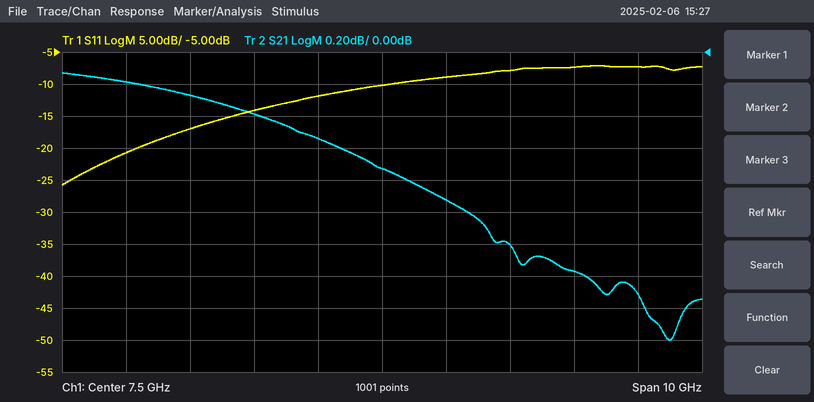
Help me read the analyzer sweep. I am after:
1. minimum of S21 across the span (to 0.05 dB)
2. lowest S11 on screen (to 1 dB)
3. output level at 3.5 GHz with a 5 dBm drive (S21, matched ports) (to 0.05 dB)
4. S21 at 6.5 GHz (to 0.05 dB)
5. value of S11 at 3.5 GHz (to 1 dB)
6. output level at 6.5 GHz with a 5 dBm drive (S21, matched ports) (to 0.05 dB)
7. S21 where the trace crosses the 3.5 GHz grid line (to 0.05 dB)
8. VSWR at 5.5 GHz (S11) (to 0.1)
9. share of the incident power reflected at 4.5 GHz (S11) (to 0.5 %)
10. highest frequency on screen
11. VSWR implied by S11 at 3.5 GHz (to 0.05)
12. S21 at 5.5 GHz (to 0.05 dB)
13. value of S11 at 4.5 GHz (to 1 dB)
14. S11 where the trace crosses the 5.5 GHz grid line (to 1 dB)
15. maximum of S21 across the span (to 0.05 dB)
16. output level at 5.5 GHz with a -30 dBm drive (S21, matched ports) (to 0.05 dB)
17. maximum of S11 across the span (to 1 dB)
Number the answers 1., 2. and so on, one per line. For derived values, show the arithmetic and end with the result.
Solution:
1. -1.80 dB
2. -26 dB
3. 5 dBm + (-0.20 dB) = 4.80 dBm
4. -0.55 dB
5. -21 dB
6. 5 dBm + (-0.55 dB) = 4.45 dBm
7. -0.20 dB
8. |Γ| = 10^(-14/20) = 0.1995; VSWR = (1 + 0.1995)/(1 − 0.1995) ≈ 1.5
9. 10^(-17/10) ≈ 2.0 %
10. 12.5 GHz
11. |Γ| = 10^(-21/20) = 0.0891; VSWR = (1 + 0.0891)/(1 − 0.0891) ≈ 1.20
12. -0.40 dB
13. -17 dB
14. -14 dB
15. -0.15 dB
16. -30 dBm + (-0.40 dB) = -30.40 dBm
17. -7 dB
